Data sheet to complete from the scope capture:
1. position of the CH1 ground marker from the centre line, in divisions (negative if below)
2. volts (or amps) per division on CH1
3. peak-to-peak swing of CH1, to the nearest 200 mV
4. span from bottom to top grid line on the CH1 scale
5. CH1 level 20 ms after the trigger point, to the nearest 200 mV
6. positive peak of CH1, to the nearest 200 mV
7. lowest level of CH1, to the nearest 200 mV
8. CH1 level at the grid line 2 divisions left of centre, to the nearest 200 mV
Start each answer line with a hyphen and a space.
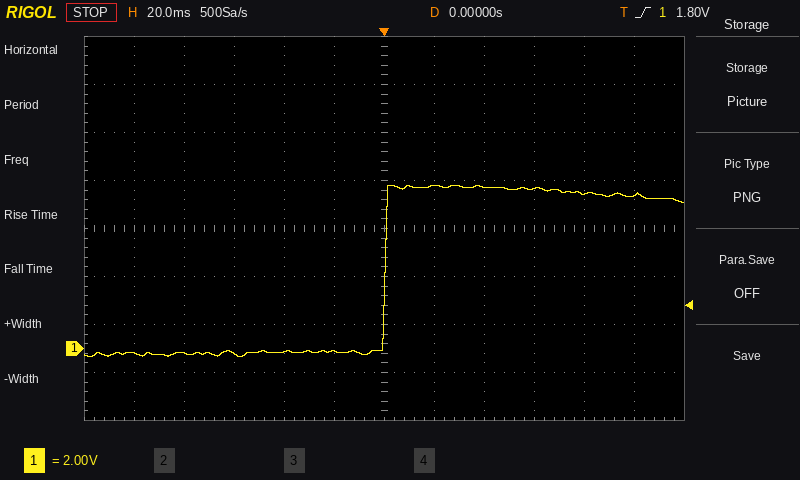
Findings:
- -2.5 div
- 2 V
- 7.2 V
- 16 V
- 6.8 V
- 6.8 V
- -400 mV
- -200 mV
